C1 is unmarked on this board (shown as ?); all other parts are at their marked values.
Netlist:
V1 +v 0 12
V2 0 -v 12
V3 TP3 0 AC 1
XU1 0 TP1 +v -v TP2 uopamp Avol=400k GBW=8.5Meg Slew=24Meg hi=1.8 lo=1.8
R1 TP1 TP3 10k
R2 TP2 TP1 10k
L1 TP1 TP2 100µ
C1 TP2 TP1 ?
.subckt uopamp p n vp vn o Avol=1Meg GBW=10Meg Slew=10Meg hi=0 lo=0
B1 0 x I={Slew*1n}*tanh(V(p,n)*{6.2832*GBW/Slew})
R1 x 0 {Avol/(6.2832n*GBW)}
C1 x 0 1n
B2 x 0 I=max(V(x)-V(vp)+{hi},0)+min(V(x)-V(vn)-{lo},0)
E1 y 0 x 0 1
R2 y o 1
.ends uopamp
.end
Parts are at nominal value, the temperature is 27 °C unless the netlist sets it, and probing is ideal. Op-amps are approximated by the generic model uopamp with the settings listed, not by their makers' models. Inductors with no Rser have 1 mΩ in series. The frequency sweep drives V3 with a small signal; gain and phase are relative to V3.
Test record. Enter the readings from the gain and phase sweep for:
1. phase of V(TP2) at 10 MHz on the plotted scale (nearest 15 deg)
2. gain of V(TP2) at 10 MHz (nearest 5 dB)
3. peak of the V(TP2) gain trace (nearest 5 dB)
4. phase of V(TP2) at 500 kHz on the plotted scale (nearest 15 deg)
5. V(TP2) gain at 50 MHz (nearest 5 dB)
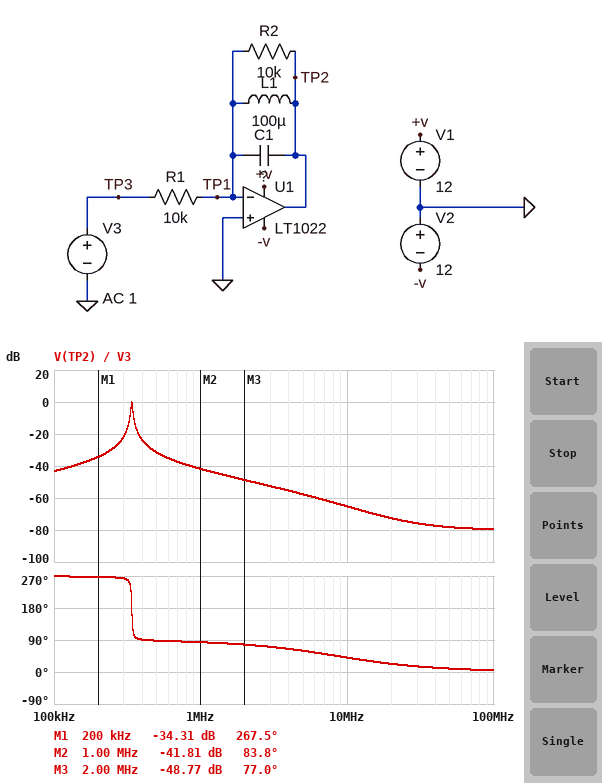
45 deg
-65 dB
0 dB
90 deg
-80 dB
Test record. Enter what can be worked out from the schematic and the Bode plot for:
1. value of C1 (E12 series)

2.2 nF
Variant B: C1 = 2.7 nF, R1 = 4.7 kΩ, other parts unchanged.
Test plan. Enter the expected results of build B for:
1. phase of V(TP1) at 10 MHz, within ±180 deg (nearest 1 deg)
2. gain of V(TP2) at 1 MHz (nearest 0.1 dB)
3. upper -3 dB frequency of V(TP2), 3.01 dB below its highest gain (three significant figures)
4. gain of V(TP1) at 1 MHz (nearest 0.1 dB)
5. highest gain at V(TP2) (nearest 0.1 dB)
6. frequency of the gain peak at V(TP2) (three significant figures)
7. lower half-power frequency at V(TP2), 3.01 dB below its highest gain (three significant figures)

-40 deg
-37.2 dB
309 kHz
-55.8 dB
6.5 dB
306 kHz
303 kHz
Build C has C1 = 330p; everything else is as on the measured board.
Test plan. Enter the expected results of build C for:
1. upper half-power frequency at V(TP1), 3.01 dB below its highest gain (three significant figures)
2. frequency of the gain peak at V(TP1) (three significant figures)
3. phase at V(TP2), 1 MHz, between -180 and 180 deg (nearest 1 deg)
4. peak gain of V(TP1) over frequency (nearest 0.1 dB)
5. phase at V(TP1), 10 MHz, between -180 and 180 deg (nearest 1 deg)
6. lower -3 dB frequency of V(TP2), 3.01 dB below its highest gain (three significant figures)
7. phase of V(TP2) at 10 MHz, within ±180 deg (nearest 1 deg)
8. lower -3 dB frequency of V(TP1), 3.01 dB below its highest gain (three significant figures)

900 kHz
874 kHz
95 deg
-19.9 dB
-48 deg
850 kHz
41 deg
851 kHz
